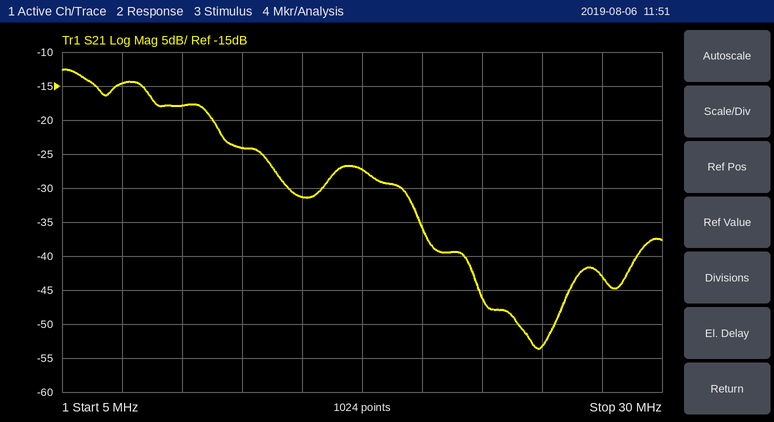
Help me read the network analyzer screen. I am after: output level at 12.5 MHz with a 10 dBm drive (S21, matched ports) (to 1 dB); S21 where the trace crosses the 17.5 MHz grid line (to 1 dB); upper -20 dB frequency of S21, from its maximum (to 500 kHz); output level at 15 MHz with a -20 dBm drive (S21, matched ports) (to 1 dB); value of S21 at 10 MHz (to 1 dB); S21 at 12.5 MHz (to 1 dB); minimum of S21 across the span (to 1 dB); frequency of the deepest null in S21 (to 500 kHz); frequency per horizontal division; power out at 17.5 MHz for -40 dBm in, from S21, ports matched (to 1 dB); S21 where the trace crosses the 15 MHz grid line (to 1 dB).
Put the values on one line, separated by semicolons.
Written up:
-14 dBm; -27 dB; 19.5 MHz; -51 dBm; -18 dB; -24 dB; -54 dB; 25.0 MHz; 2.5 MHz; -67 dBm; -31 dB
